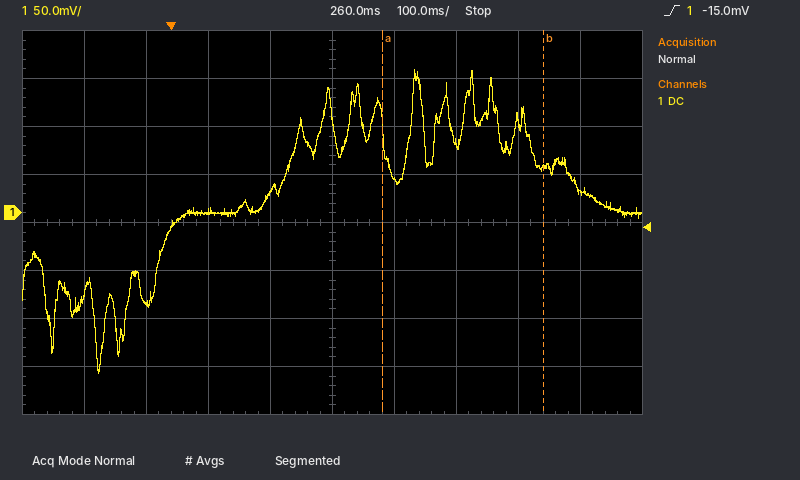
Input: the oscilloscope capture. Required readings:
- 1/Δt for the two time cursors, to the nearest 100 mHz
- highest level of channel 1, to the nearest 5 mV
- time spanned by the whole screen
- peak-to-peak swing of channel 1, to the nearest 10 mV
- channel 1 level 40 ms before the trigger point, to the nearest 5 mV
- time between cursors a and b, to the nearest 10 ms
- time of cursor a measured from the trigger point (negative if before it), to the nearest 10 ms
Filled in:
3.8 Hz
150 mV
1 s
320 mV
-95 mV
260 ms
+340 ms
